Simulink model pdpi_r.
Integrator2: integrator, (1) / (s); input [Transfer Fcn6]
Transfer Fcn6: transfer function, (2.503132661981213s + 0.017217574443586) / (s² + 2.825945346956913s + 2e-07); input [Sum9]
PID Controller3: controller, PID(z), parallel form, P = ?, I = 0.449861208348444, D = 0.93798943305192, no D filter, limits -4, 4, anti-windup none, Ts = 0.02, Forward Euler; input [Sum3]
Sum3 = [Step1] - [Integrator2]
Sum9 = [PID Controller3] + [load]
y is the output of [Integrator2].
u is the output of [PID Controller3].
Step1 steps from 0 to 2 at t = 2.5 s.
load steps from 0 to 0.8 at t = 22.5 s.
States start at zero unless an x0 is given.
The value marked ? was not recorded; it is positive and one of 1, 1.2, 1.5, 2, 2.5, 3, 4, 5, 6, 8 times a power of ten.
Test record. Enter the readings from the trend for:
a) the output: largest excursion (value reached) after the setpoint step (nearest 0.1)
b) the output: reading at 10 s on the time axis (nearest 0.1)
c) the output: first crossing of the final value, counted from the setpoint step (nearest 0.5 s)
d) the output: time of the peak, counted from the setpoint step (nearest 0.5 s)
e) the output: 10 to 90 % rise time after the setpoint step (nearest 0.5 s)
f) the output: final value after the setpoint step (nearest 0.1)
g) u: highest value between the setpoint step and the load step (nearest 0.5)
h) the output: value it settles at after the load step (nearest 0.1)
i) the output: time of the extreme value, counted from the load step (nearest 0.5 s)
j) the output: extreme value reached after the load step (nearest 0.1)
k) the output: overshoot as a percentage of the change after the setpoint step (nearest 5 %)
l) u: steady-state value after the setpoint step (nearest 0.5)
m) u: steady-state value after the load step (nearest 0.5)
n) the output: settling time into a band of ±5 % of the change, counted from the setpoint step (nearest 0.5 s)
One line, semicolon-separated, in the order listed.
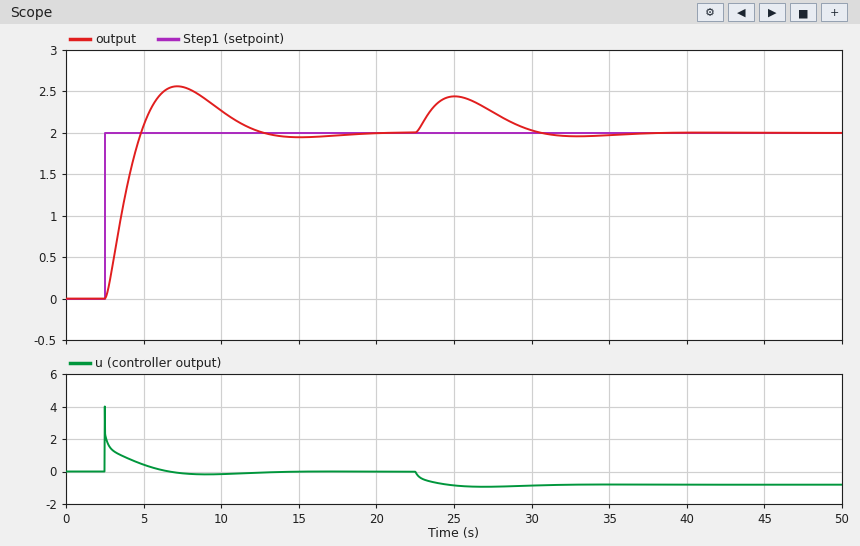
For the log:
2.6; 2.3; 2.5 s; 4.5 s; 1.5 s; 2.0; 4.0; 2.0; 2.5 s; 2.4; 30 %; 0.0; -1.0; 9.0 s
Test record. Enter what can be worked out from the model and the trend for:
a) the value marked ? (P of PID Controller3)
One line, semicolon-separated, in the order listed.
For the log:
1.2
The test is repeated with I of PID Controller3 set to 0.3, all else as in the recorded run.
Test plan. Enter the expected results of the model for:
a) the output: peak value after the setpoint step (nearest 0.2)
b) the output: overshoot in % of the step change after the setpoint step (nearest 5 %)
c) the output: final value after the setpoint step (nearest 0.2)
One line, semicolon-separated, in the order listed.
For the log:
2.4; 20 %; 2.0
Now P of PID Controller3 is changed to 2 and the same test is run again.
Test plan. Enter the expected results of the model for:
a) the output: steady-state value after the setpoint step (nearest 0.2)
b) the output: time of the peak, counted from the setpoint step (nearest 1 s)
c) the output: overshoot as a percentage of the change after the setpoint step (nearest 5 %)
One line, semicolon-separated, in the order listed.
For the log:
2.0; 4 s; 15 %
